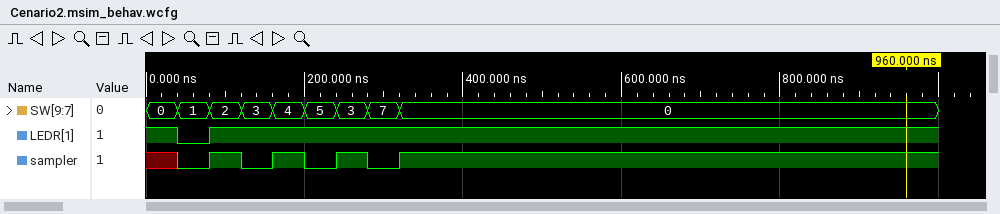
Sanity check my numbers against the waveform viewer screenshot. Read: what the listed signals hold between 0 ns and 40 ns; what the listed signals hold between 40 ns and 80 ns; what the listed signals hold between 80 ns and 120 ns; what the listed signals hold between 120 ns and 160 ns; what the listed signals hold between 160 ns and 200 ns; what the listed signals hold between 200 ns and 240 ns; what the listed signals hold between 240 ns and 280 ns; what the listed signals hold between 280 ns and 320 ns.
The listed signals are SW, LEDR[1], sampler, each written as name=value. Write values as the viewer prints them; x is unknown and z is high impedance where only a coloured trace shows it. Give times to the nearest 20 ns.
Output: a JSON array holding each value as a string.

["SW=0, LEDR[1]=1, sampler=x", "SW=1, LEDR[1]=0, sampler=0", "SW=2, LEDR[1]=1, sampler=1", "SW=3, LEDR[1]=1, sampler=0", "SW=4, LEDR[1]=1, sampler=1", "SW=5, LEDR[1]=1, sampler=0", "SW=3, LEDR[1]=1, sampler=1", "SW=7, LEDR[1]=1, sampler=0"]
